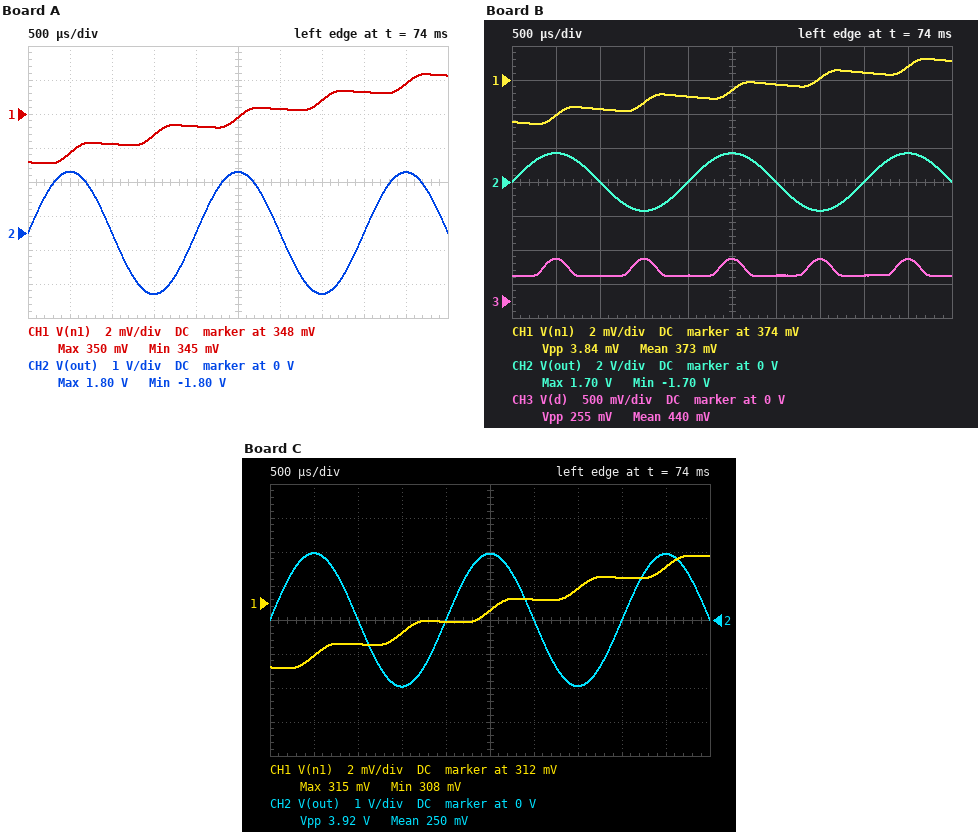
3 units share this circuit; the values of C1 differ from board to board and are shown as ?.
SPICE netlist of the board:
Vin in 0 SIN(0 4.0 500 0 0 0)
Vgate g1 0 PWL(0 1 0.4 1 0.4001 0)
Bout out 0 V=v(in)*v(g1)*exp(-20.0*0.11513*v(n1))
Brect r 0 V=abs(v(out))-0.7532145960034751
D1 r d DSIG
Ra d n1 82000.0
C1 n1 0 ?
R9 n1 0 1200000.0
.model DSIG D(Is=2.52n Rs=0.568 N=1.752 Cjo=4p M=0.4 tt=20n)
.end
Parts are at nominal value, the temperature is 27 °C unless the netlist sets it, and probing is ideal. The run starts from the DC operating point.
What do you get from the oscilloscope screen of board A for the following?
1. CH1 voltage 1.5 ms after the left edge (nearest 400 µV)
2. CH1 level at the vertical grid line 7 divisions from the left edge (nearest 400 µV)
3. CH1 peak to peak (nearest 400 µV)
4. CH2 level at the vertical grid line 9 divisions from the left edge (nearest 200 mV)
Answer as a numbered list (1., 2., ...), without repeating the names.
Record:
1. 346.8 mV
2. 348.8 mV
3. 5.2 mV
4. 1.8 V
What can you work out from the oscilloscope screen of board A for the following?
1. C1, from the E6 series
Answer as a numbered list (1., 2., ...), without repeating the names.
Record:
1. 1 µF
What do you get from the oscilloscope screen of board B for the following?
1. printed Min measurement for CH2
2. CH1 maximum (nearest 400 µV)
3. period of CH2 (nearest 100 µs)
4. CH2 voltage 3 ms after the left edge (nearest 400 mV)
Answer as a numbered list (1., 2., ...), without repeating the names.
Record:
1. -1.70 V
2. 375.2 mV
3. 2.0 ms
4. 0 V
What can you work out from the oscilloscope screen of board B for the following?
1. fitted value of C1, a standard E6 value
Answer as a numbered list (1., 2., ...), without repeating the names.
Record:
1. 680 nF
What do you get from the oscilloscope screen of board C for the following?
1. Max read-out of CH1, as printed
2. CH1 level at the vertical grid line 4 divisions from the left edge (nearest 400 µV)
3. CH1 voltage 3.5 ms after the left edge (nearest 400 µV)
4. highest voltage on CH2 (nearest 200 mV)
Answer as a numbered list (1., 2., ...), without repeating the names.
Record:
1. 315 mV
2. 310.8 mV
3. 312.8 mV
4. 2.0 V
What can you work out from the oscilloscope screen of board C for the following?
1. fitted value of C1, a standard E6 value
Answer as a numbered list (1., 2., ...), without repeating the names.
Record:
1. 1.5 µF
